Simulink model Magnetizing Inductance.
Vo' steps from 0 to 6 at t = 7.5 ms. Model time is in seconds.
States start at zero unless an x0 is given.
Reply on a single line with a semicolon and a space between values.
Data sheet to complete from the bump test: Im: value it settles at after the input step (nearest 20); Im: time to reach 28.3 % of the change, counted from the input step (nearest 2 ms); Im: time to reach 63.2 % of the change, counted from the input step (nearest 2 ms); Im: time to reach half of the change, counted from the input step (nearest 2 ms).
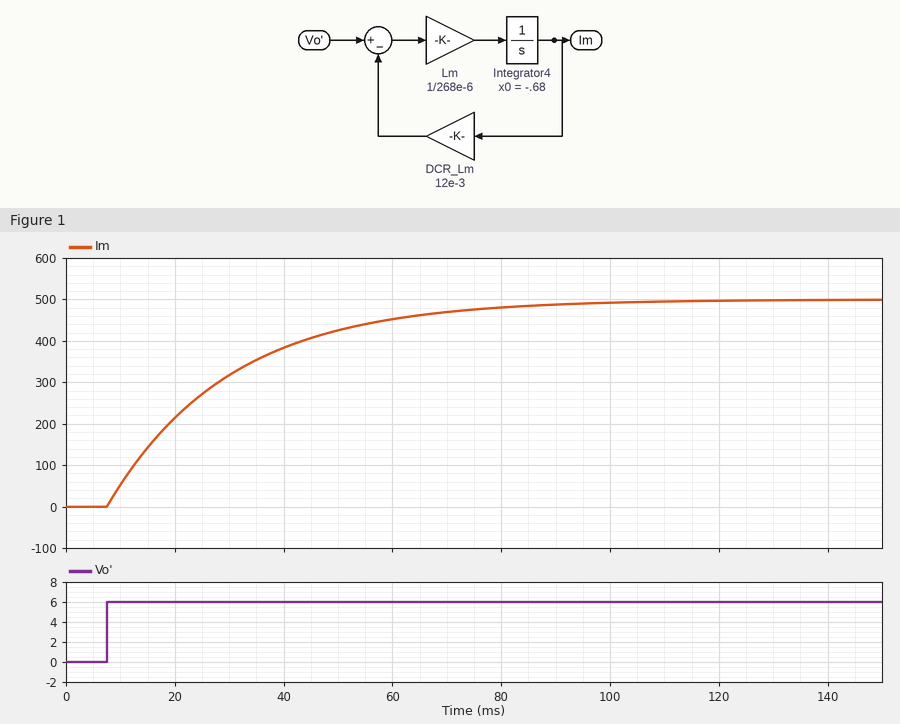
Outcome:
500; 8 ms; 22 ms; 16 ms
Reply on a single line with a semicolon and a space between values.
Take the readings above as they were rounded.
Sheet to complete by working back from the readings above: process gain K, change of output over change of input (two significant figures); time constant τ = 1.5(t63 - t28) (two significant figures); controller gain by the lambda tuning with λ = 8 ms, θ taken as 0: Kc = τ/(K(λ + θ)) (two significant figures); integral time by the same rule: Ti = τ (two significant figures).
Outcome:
83; 21 ms; 0.032; 21 ms
